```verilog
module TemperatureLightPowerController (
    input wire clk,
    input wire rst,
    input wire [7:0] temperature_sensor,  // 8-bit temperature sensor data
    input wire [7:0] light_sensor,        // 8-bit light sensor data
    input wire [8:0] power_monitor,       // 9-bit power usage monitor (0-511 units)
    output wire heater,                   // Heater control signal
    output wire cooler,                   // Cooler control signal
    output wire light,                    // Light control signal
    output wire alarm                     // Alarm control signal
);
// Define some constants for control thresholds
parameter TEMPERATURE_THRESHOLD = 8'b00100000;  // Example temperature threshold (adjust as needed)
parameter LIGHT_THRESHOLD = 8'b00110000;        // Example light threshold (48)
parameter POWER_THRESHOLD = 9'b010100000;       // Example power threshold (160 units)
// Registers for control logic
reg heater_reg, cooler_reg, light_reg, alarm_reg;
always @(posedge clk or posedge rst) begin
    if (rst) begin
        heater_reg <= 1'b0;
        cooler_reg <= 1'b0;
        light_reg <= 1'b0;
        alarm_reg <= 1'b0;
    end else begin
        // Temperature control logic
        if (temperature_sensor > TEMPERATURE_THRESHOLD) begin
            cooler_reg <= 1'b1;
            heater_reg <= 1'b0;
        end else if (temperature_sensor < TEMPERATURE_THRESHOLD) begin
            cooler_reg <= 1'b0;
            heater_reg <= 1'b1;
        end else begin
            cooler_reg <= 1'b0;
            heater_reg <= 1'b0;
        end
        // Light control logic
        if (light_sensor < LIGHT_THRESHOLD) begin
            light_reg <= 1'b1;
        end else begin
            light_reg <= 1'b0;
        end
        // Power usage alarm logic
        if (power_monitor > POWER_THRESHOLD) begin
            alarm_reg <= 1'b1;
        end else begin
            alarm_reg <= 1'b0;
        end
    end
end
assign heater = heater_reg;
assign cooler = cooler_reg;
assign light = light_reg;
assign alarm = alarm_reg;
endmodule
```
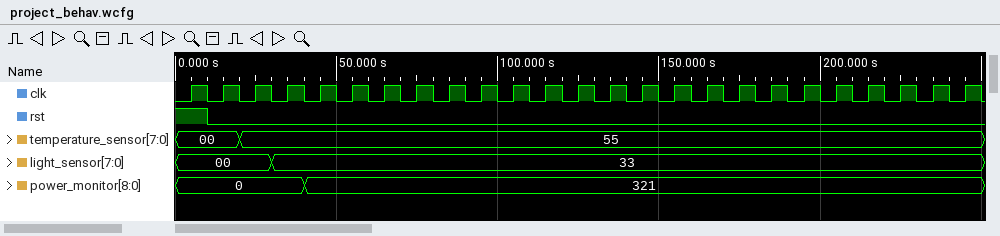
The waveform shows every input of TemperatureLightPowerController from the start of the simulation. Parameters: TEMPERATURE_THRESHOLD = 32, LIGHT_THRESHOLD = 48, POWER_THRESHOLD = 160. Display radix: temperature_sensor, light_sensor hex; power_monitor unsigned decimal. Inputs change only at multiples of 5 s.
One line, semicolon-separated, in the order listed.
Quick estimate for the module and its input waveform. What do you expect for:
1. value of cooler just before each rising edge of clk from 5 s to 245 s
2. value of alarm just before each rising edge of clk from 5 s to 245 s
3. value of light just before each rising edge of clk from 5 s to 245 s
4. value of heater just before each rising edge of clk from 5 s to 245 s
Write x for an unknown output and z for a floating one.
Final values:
0 0 0 1 1 1 1 1 1 1 1 1 1 1 1 1 1 1 1 1 1 1 1 1 1; 0 0 0 0 0 1 1 1 1 1 1 1 1 1 1 1 1 1 1 1 1 1 1 1 1; 0 0 1 1 0 0 0 0 0 0 0 0 0 0 0 0 0 0 0 0 0 0 0 0 0; 0 0 1 0 0 0 0 0 0 0 0 0 0 0 0 0 0 0 0 0 0 0 0 0 0
